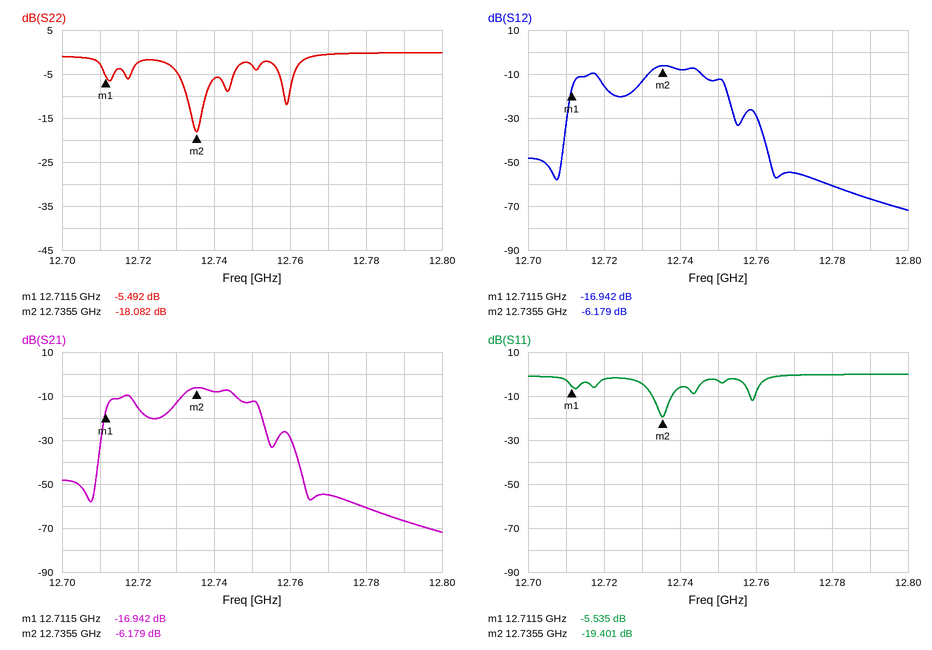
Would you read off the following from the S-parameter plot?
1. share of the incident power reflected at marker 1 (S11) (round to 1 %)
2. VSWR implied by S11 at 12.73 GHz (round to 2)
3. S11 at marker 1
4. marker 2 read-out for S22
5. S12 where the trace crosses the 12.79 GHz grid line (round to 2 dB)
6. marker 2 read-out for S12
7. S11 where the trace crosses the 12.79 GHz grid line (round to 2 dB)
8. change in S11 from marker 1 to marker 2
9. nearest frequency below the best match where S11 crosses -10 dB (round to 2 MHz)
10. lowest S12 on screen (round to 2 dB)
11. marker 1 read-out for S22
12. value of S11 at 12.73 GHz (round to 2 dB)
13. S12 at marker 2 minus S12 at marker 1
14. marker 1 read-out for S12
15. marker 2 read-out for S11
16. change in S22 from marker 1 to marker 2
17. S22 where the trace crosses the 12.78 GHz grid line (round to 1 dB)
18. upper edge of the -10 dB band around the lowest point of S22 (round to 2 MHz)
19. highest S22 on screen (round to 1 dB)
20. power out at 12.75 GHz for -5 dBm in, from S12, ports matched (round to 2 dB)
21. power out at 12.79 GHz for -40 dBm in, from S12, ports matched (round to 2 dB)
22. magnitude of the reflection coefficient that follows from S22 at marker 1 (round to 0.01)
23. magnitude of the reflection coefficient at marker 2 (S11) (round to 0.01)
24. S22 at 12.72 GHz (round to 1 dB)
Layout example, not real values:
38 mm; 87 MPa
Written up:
28 %; 4; -5.535 dB; -18.082 dB; -66 dB; -6.179 dB; 0 dB; -13.866 dB; 12.732 GHz; -72 dB; -5.492 dB; -4 dB; 10.763 dB; -16.942 dB; -19.401 dB; -12.590 dB; 0 dB; 12.738 GHz; 0 dB; -18 dBm; -106 dBm; 0.53; 0.11; -2 dB
